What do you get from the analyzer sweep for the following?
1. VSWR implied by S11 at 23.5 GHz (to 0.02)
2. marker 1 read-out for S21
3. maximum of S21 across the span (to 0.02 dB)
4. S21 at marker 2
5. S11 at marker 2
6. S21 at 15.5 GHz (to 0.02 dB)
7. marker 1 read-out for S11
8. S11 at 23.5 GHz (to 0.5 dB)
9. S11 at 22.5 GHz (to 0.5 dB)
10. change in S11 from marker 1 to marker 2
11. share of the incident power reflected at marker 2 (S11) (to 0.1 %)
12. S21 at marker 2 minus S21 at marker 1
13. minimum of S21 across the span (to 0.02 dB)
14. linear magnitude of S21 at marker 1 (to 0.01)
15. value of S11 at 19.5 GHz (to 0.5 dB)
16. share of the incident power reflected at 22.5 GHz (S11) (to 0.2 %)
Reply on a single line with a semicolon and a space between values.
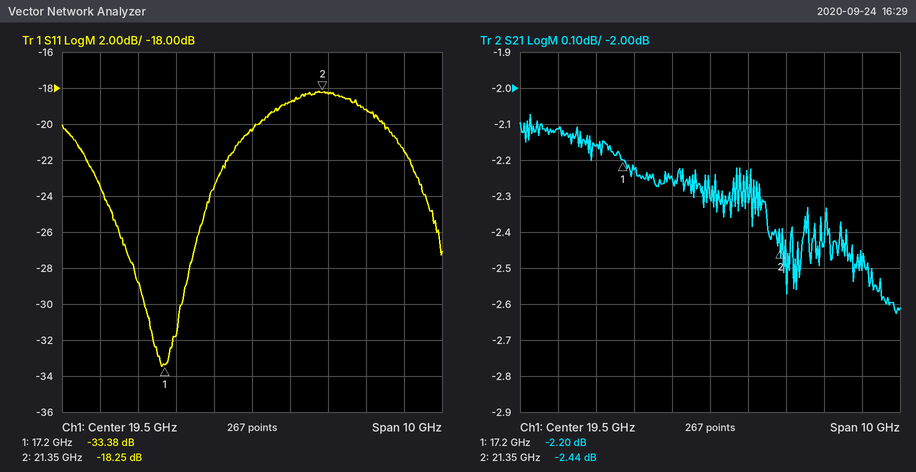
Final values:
1.18; -2.20 dB; -2.08 dB; -2.44 dB; -18.25 dB; -2.12 dB; -33.38 dB; -21.5 dB; -19.0 dB; 15.13 dB; 1.5 %; -0.24 dB; -2.62 dB; 0.78; -20.5 dB; 1.2 %
